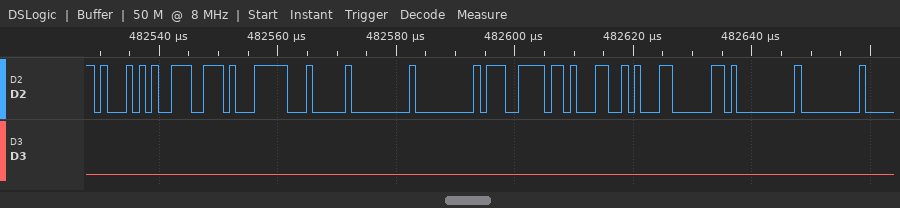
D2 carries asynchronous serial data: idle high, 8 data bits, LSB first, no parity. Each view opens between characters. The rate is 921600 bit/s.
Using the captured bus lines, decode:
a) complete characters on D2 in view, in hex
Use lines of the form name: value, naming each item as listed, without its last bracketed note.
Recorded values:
complete characters on D2 in view, in hex: 51, CE, F1, 04, 00, 00, E7, 8B, 8A, 60, 00, 00
